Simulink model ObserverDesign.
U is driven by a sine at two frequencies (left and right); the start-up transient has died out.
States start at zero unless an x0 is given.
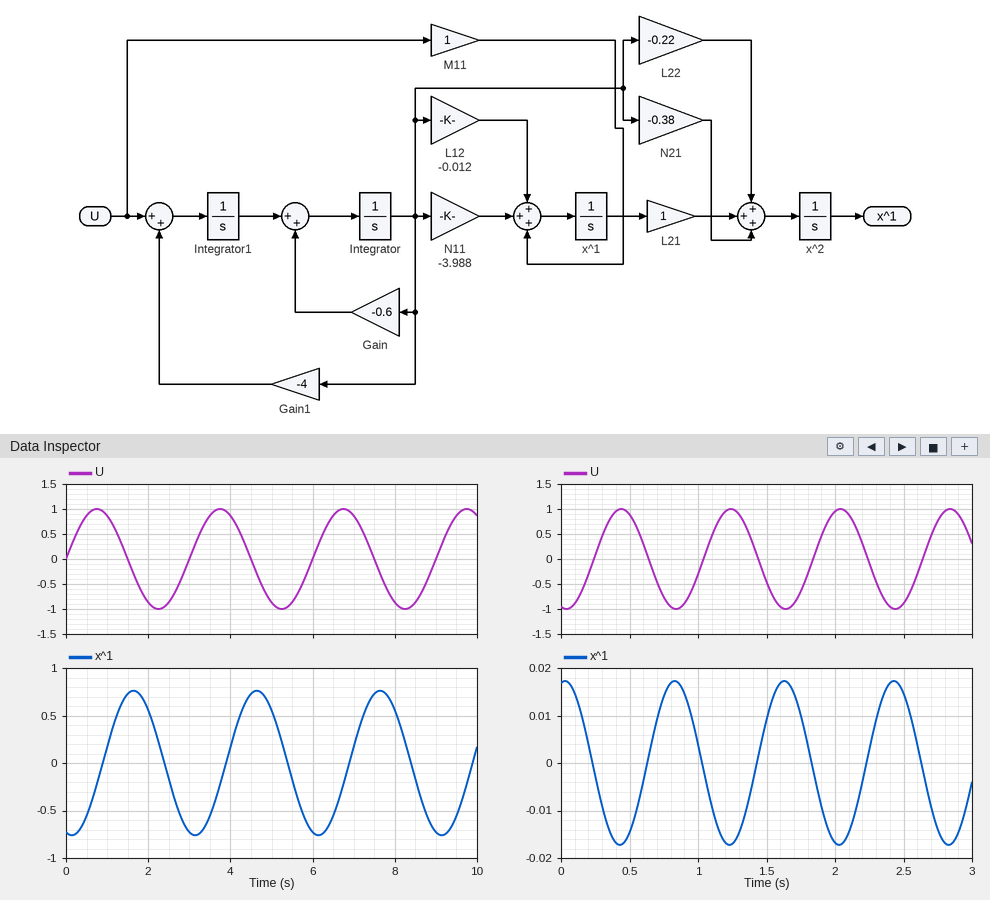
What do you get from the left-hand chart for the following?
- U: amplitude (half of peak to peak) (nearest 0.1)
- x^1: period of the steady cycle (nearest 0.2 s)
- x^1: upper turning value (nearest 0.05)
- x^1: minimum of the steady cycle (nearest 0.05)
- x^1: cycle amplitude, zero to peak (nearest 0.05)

1.0
3.0 s
0.75
-0.75
0.75
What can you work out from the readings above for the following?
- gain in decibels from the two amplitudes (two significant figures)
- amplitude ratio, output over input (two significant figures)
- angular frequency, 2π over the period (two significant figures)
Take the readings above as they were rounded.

-2.5 dB
0.75
2.1 rad/s
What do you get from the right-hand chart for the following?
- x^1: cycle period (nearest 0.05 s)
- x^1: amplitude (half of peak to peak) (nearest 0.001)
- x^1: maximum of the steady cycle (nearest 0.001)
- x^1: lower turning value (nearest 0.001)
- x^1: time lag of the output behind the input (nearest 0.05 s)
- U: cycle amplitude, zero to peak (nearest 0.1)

0.80 s
0.017
0.017
-0.017
0.40 s
1.0
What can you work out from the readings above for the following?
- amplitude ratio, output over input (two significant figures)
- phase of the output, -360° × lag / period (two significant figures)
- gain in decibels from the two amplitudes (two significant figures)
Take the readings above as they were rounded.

0.017
-180°
-35 dB
